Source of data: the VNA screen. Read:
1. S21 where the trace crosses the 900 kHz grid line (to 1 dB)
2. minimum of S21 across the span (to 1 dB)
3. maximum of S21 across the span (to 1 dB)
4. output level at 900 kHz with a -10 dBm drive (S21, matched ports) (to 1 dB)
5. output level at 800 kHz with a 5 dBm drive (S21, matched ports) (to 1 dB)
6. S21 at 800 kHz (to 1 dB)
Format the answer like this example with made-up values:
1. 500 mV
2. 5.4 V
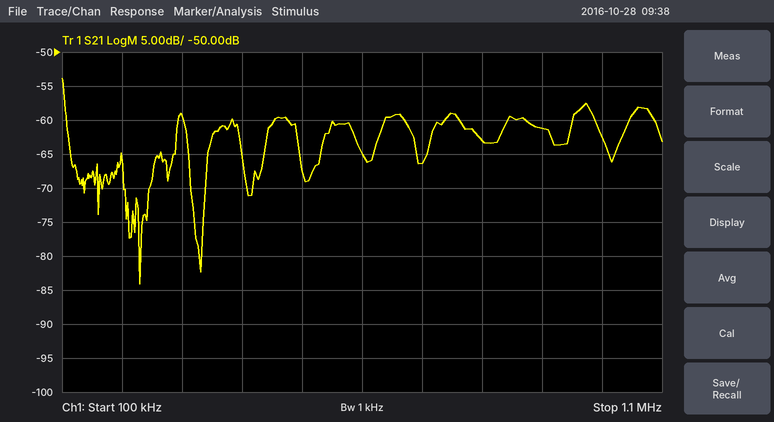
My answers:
1. -61 dB
2. -84 dB
3. -54 dB
4. -71 dBm
5. -58 dBm
6. -63 dB
